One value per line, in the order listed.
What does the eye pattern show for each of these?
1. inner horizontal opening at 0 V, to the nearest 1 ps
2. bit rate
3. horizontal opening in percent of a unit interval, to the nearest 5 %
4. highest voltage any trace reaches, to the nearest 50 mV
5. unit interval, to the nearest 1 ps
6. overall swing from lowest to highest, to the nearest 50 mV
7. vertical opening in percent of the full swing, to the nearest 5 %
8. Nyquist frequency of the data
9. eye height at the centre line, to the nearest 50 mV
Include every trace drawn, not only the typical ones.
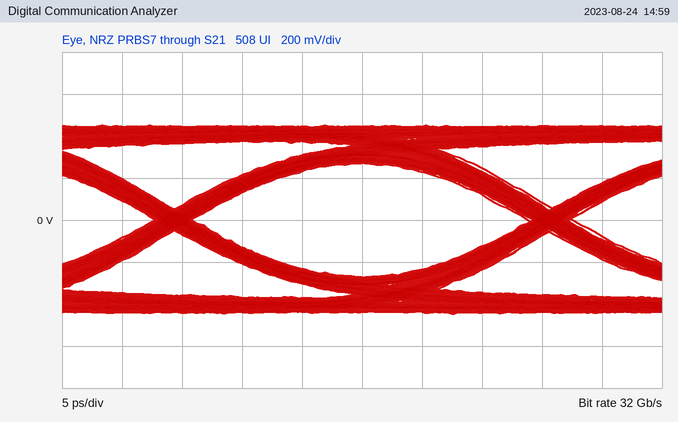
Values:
28 ps
32 Gb/s
90 %
450 mV
31 ps
900 mV
60 %
16 GHz
550 mV
